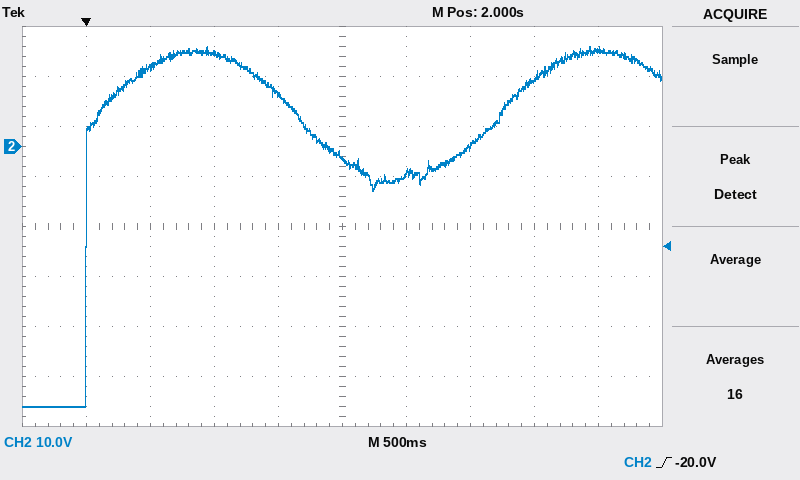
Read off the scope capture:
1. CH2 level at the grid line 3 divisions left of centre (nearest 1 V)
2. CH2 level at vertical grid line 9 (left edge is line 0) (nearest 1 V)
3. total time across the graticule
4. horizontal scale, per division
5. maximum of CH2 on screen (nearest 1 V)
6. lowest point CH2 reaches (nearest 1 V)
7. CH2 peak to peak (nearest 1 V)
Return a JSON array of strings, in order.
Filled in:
["16 V", "19 V", "5 s", "500 ms", "20 V", "-52 V", "72 V"]
